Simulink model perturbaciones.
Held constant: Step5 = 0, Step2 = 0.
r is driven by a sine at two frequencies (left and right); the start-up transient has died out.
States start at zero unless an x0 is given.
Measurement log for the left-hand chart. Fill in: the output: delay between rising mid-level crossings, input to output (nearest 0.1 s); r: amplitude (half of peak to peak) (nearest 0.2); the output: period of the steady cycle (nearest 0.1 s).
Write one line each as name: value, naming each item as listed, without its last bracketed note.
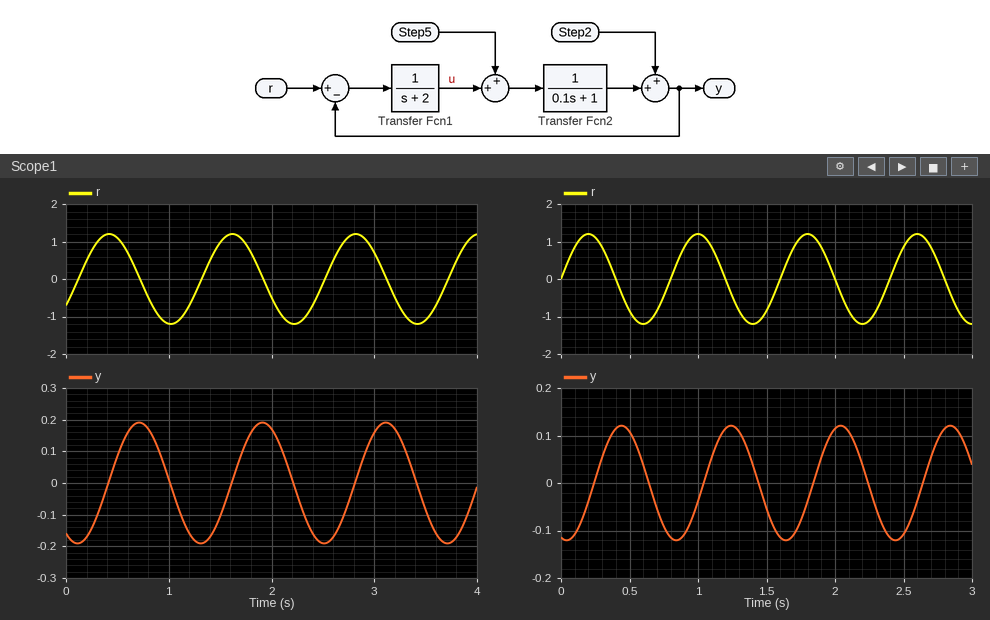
the output: delay between rising mid-level crossings, input to output: 0.3 s
r: amplitude (half of peak to peak): 1.2
the output: period of the steady cycle: 1.2 s
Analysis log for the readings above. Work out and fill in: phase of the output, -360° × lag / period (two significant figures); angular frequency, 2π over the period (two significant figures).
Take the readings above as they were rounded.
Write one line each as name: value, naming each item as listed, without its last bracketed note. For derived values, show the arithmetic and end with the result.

phase of the output, -360° × lag / period: -360 × 0.3 / 1.2 = -90°
angular frequency, 2π over the period: 2π / 1.2 = 5.2 rad/s
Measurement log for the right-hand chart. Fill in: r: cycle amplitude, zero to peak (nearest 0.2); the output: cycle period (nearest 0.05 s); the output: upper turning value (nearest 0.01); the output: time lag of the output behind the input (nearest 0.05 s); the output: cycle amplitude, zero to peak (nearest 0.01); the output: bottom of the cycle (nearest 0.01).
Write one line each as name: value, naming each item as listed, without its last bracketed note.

r: cycle amplitude, zero to peak: 1.2
the output: cycle period: 0.80 s
the output: upper turning value: 0.12
the output: time lag of the output behind the input: 0.25 s
the output: cycle amplitude, zero to peak: 0.12
the output: bottom of the cycle: -0.12
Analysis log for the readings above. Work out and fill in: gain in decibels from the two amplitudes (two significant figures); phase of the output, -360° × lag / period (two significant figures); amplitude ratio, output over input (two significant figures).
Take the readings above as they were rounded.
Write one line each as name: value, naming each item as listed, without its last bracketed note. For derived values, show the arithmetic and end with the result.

gain in decibels from the two amplitudes: 20 log10(0.12 / 1.2) = -20 dB
phase of the output, -360° × lag / period: -360 × 0.25 / 0.8 = -110°
amplitude ratio, output over input: 0.12 / 1.2 = 0.10
